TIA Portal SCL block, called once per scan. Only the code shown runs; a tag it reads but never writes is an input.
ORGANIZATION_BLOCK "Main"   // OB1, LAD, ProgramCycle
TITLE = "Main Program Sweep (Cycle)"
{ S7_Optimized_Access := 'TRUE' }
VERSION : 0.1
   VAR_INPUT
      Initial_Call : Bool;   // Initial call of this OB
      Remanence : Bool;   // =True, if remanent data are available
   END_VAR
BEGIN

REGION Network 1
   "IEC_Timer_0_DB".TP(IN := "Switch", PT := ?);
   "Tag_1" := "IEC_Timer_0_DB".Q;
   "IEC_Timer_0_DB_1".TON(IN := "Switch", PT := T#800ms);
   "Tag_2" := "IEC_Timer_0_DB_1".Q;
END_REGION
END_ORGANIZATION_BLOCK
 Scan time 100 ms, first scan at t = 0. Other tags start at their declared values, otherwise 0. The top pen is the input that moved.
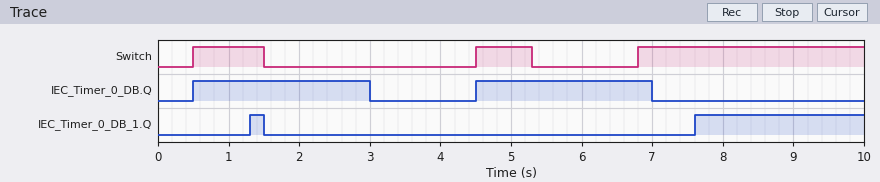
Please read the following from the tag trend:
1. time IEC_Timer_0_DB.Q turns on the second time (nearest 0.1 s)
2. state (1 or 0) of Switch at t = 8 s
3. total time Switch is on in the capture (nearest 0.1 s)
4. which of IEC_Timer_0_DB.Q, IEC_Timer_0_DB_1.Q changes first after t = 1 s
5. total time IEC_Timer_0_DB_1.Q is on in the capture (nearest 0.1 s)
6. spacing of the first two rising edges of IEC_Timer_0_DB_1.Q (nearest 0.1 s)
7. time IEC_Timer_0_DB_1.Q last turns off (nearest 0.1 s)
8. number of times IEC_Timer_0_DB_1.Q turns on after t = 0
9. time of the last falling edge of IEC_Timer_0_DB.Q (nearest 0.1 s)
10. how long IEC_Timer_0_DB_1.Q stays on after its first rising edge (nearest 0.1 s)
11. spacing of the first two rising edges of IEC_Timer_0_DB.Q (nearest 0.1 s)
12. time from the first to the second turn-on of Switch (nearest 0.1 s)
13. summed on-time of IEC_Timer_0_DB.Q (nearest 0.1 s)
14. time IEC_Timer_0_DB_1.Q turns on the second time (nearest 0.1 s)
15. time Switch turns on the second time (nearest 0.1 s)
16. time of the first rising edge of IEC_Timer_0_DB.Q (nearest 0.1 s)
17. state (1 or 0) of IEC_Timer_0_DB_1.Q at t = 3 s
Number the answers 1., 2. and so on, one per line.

1. 4.5 s
2. 1
3. 5.0 s
4. IEC_Timer_0_DB_1.Q
5. 2.6 s
6. 6.3 s
7. 1.5 s
8. 2
9. 7.0 s
10. 0.2 s
11. 4.0 s
12. 4.0 s
13. 5.0 s
14. 7.6 s
15. 4.5 s
16. 0.5 s
17. 0
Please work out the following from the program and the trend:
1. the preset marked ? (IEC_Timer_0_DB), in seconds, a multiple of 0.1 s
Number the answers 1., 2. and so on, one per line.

1. 2.5 s
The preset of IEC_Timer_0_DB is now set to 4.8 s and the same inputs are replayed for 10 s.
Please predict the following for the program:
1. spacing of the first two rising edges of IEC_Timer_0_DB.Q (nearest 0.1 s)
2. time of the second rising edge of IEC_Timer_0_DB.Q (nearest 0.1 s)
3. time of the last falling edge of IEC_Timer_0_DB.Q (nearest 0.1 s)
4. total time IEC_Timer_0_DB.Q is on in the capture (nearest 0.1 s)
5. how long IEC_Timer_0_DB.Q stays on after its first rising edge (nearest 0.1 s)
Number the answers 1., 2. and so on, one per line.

1. 6.3 s
2. 6.8 s
3. 5.3 s
4. 8.0 s
5. 4.8 s
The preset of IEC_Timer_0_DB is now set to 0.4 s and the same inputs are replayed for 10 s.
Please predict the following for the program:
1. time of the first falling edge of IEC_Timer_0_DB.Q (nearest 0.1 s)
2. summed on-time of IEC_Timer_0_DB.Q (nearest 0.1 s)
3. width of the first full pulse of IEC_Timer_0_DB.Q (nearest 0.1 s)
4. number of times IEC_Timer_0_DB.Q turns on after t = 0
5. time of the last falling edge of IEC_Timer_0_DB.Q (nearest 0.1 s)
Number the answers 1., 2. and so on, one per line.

1. 0.9 s
2. 1.2 s
3. 0.4 s
4. 3
5. 7.2 s
